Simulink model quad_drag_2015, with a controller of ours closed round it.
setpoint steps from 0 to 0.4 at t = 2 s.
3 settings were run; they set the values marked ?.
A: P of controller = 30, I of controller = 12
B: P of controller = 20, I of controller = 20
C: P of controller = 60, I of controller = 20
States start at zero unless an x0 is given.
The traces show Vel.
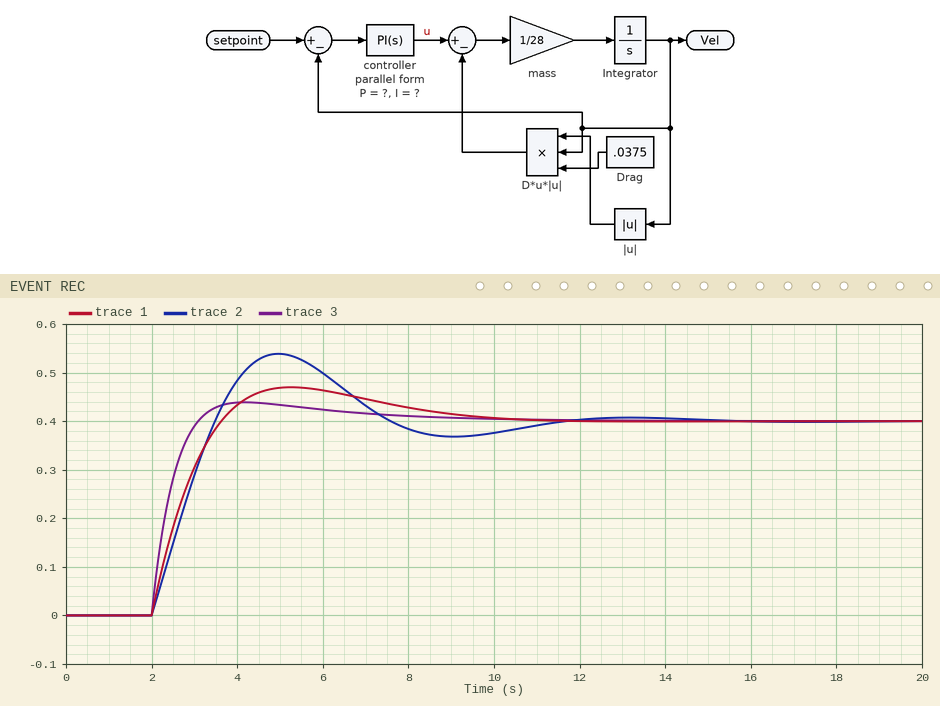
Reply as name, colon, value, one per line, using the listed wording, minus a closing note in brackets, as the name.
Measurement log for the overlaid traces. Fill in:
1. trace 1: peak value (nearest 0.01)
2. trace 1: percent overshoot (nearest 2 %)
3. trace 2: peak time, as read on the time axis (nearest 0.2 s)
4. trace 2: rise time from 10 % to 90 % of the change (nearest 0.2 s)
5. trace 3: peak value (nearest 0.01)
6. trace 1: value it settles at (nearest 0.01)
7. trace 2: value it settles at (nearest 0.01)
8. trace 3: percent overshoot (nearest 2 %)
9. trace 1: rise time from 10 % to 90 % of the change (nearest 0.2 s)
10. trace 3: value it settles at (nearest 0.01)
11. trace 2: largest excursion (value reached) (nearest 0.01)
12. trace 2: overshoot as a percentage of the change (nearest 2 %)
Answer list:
trace 1: peak value: 0.47
trace 1: percent overshoot: 18 %
trace 2: peak time, as read on the time axis: 5.0 s
trace 2: rise time from 10 % to 90 % of the change: 1.2 s
trace 3: peak value: 0.44
trace 1: value it settles at: 0.40
trace 2: value it settles at: 0.40
trace 3: percent overshoot: 10 %
trace 1: rise time from 10 % to 90 % of the change: 1.2 s
trace 3: value it settles at: 0.40
trace 2: largest excursion (value reached): 0.54
trace 2: overshoot as a percentage of the change: 34 %
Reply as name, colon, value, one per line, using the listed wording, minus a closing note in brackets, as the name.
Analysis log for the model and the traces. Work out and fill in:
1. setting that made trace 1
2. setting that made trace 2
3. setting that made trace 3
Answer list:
setting that made trace 1: A
setting that made trace 2: B
setting that made trace 3: C
